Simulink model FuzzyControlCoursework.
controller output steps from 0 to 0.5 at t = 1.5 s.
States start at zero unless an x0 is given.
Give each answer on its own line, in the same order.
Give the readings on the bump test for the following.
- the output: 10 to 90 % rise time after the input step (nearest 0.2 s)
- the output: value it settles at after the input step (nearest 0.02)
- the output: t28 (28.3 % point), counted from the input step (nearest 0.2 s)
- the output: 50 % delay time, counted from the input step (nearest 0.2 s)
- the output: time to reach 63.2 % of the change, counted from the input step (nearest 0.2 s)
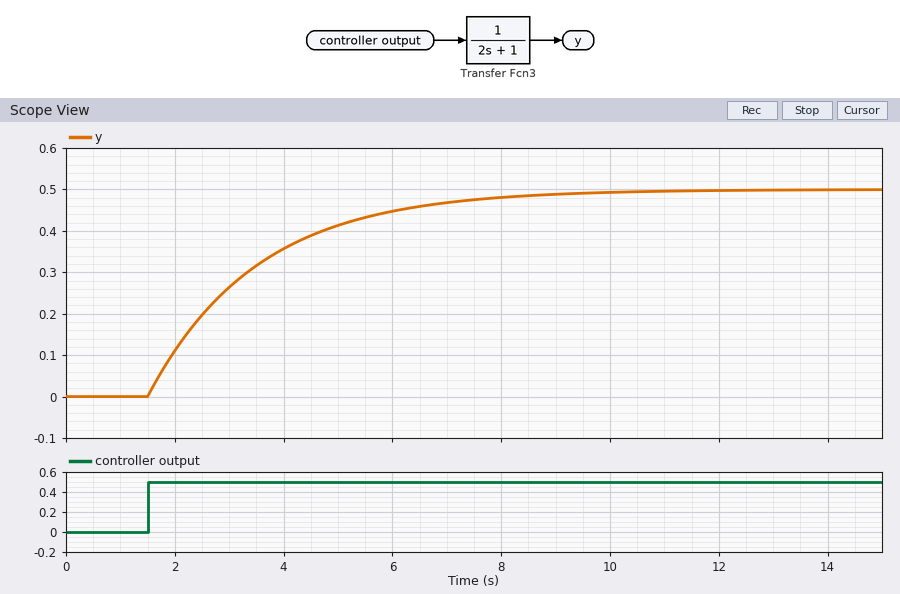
4.4 s
0.50
0.6 s
1.4 s
2.0 s
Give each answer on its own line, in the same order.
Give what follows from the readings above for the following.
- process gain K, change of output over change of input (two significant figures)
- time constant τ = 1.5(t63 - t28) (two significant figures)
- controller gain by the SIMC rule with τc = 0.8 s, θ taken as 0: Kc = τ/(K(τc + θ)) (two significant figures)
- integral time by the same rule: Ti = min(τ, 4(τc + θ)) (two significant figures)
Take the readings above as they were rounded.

1.0
2.1 s
2.6
2.1 s
